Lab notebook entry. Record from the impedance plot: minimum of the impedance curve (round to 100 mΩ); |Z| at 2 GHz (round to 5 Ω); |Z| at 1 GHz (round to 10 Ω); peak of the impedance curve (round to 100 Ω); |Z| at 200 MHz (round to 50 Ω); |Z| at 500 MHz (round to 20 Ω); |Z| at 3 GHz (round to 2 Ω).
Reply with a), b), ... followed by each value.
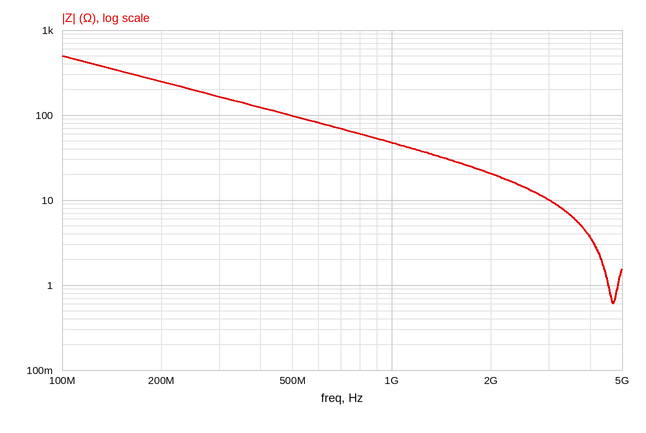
a) 600 mΩ
b) 20 Ω
c) 50 Ω
d) 500 Ω
e) 250 Ω
f) 100 Ω
g) 10 Ω
